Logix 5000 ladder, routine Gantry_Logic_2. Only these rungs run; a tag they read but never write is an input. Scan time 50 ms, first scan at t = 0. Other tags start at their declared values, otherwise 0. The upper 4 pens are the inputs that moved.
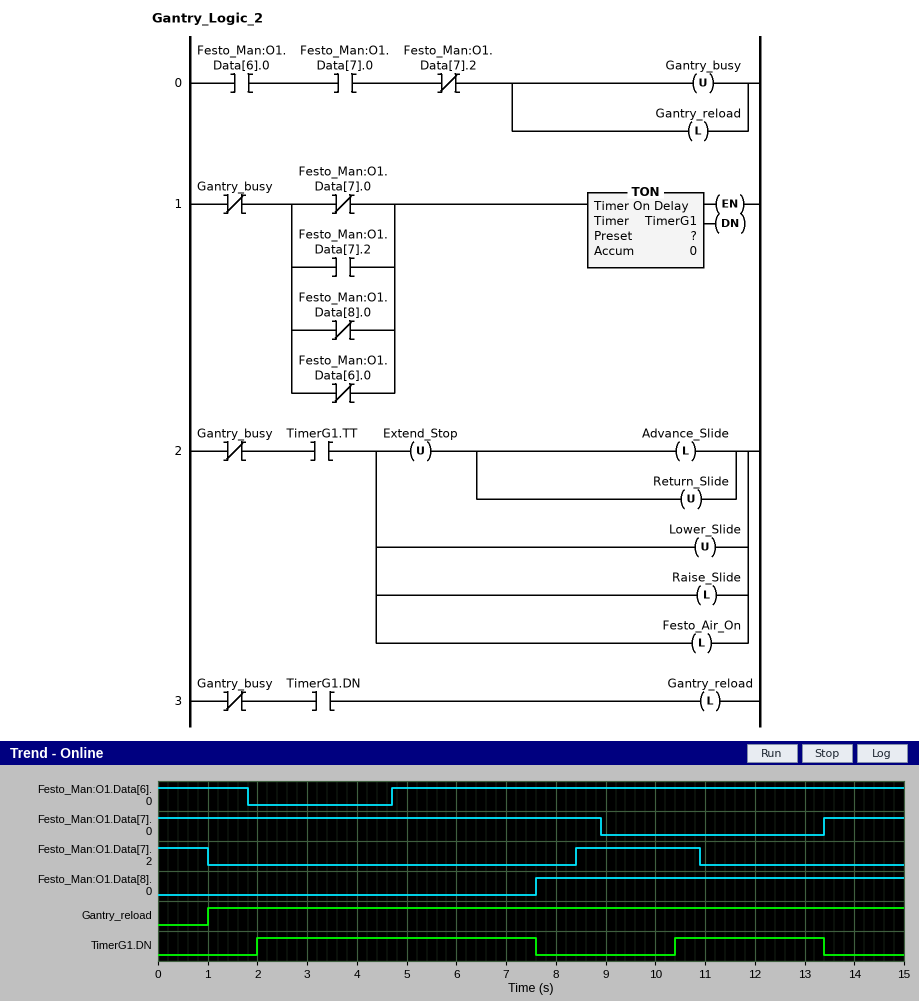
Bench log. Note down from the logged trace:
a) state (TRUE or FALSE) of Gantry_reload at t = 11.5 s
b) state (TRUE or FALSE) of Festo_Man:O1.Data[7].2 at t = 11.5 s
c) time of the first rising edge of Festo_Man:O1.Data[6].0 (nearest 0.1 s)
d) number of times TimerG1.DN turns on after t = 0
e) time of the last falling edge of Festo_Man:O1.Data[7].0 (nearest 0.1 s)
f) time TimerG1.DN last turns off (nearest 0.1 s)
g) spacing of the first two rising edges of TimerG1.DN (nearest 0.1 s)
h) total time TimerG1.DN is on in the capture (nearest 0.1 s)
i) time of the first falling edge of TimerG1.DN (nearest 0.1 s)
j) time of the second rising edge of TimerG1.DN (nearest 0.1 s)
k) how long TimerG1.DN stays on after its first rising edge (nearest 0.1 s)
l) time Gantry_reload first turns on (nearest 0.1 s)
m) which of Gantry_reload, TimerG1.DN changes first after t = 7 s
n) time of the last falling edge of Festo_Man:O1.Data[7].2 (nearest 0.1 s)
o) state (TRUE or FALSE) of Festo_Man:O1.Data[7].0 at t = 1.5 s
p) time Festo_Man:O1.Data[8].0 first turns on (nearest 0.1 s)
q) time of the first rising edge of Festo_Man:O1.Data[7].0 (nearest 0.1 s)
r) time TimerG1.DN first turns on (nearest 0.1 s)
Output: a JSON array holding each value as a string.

["TRUE", "FALSE", "4.7 s", "2", "8.9 s", "13.4 s", "8.4 s", "8.6 s", "7.6 s", "10.4 s", "5.6 s", "1.0 s", "TimerG1.DN", "10.9 s", "TRUE", "7.6 s", "13.4 s", "2.0 s"]
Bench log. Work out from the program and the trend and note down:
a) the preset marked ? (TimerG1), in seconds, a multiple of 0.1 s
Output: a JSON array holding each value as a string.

["2.0 s"]
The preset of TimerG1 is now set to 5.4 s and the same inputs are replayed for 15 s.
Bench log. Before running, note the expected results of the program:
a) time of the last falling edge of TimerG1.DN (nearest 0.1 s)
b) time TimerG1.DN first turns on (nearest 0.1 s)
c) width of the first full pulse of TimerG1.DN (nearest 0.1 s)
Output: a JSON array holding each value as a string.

["7.6 s", "5.4 s", "2.2 s"]
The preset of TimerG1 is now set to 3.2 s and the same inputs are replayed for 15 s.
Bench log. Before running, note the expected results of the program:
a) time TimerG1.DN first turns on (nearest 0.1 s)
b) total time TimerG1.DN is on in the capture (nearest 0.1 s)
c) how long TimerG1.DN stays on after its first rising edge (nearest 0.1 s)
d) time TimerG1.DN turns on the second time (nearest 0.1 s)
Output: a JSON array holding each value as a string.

["3.2 s", "6.2 s", "4.4 s", "11.6 s"]
